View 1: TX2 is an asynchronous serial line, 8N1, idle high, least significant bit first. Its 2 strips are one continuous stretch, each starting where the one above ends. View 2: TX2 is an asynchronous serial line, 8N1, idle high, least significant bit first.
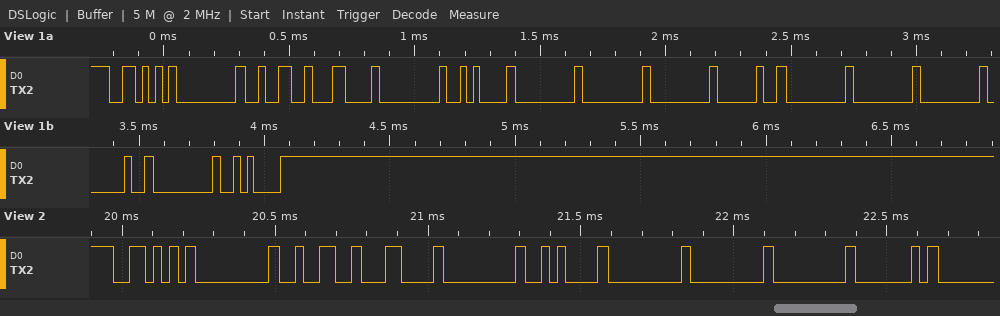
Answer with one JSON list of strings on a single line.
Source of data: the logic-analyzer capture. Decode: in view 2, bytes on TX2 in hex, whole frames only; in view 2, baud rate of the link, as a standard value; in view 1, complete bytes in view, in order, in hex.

["0x56 0x00 0x32 0x0C 0x00 0x0A 0x00 0x00 0x00 0x40", "38400 baud", "56 00 32 0C 00 0A 00 00 00 20 00 00 00 20 00 0A"]
